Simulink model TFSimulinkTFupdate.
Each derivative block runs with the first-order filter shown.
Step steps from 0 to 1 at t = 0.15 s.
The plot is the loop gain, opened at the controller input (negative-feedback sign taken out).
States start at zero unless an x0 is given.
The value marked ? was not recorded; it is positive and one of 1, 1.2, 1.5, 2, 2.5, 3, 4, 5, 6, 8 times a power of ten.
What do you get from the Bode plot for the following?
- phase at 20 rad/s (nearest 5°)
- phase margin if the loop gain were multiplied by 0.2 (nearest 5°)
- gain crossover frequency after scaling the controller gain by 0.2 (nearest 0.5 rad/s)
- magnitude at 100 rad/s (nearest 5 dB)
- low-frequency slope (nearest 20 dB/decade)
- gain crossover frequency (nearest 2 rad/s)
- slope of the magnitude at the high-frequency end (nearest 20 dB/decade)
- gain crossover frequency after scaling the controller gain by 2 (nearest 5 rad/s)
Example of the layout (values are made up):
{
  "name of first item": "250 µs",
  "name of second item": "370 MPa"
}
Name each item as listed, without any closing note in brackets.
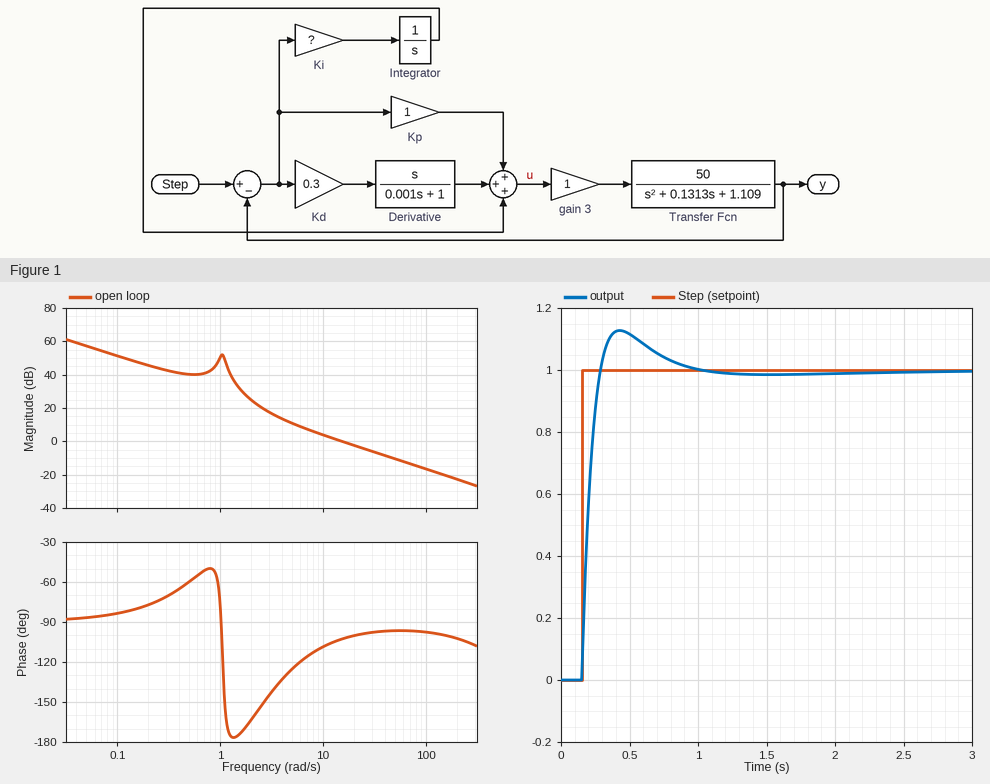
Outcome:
{
  "phase at 20 rad/s": "-100°",
  "phase margin if the loop gain were multiplied by 0.2": "45°",
  "gain crossover frequency after scaling the controller gain by 0.2": "4.0 rad/s",
  "magnitude at 100 rad/s": "-15 dB",
  "low-frequency slope": "-20 dB/decade",
  "gain crossover frequency": "16 rad/s",
  "slope of the magnitude at the high-frequency end": "-20 dB/decade",
  "gain crossover frequency after scaling the controller gain by 2": "30 rad/s"
}
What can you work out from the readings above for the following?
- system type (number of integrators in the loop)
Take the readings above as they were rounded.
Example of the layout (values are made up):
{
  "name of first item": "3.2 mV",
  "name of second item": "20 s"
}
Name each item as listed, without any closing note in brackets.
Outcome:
{
  "system type": "1"
}
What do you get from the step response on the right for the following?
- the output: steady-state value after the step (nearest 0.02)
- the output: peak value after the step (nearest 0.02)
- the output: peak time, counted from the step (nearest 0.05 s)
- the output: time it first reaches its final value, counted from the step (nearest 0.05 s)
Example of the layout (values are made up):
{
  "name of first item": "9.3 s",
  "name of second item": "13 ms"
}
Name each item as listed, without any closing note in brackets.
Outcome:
{
  "the output: steady-state value after the step": "1.00",
  "the output: peak value after the step": "1.12",
  "the output: peak time, counted from the step": "0.30 s",
  "the output: time it first reaches its final value, counted from the step": "0.15 s"
}
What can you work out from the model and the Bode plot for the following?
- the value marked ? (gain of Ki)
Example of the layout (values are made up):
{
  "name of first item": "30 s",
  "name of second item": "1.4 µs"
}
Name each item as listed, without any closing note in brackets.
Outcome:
{
  "the value marked ?": "0.8"
}
